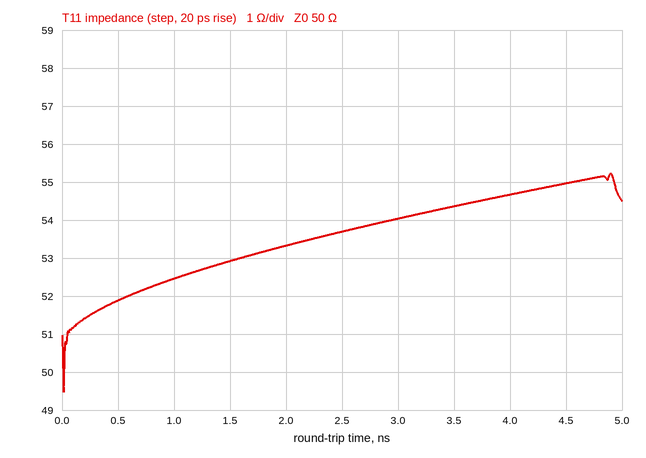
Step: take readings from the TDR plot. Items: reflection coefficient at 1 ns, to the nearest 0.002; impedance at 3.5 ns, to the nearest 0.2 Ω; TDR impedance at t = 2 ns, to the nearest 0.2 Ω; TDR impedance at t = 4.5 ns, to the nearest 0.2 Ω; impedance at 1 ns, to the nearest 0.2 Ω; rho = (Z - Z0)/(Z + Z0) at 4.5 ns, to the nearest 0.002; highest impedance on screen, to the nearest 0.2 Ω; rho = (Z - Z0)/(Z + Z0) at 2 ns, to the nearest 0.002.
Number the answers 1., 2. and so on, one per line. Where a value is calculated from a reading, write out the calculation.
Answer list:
1. (52.4 − 50)/(52.4 + 50) ≈ +0.0234, so +0.024 to the nearest 0.002
2. 54.4 Ω
3. 53.4 Ω
4. 55.0 Ω
5. 52.4 Ω
6. (55 − 50)/(55 + 50) ≈ +0.048
7. 55.2 Ω
8. (53.4 − 50)/(53.4 + 50) ≈ +0.0329, so +0.032 to the nearest 0.002
